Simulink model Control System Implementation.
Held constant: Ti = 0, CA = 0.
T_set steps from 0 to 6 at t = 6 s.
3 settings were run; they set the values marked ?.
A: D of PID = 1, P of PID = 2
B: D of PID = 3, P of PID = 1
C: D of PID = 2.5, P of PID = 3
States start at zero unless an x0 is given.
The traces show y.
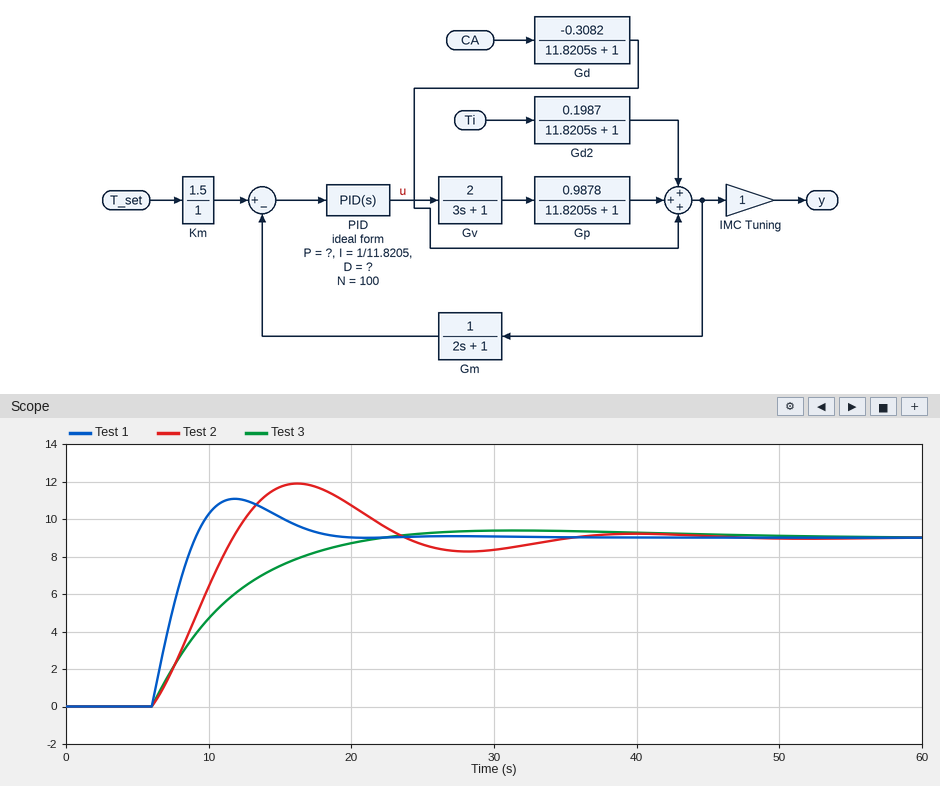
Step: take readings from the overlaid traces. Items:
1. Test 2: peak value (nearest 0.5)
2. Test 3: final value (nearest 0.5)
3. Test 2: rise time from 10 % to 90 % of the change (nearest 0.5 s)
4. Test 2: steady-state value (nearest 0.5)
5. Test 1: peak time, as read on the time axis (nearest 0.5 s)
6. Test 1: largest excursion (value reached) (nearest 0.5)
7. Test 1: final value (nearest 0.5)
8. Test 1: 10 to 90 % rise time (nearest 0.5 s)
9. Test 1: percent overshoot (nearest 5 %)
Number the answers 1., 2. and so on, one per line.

1. 12.0
2. 9.0
3. 4.5 s
4. 9.0
5. 12.0 s
6. 11.0
7. 9.0
8. 2.5 s
9. 25 %
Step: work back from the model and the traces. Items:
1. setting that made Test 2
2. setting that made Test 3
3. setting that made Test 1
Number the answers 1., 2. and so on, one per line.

1. A
2. B
3. C
